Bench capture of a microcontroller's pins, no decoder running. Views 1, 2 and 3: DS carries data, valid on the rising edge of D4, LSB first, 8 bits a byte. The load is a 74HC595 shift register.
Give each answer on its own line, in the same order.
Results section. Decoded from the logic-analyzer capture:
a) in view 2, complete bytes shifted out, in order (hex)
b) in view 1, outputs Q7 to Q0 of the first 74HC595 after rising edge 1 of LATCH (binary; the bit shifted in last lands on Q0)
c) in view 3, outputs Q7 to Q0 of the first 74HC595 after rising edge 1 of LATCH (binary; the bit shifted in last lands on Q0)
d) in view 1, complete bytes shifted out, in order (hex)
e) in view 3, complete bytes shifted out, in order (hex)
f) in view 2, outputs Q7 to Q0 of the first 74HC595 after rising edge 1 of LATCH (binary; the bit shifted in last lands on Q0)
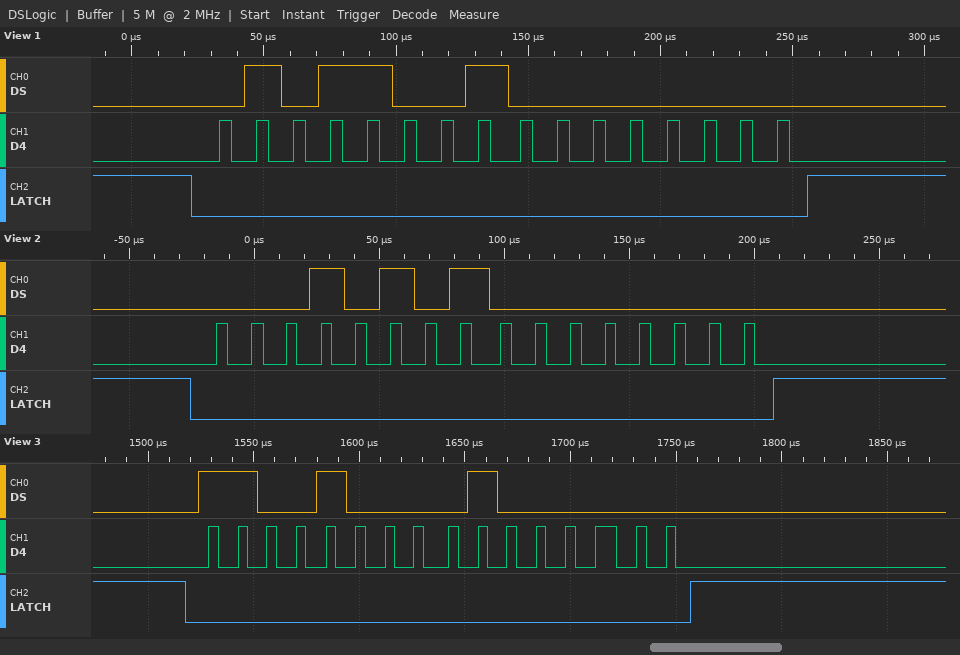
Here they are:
0xA8 0x00
00000000
01000000
9A 00
13 02
00000000
